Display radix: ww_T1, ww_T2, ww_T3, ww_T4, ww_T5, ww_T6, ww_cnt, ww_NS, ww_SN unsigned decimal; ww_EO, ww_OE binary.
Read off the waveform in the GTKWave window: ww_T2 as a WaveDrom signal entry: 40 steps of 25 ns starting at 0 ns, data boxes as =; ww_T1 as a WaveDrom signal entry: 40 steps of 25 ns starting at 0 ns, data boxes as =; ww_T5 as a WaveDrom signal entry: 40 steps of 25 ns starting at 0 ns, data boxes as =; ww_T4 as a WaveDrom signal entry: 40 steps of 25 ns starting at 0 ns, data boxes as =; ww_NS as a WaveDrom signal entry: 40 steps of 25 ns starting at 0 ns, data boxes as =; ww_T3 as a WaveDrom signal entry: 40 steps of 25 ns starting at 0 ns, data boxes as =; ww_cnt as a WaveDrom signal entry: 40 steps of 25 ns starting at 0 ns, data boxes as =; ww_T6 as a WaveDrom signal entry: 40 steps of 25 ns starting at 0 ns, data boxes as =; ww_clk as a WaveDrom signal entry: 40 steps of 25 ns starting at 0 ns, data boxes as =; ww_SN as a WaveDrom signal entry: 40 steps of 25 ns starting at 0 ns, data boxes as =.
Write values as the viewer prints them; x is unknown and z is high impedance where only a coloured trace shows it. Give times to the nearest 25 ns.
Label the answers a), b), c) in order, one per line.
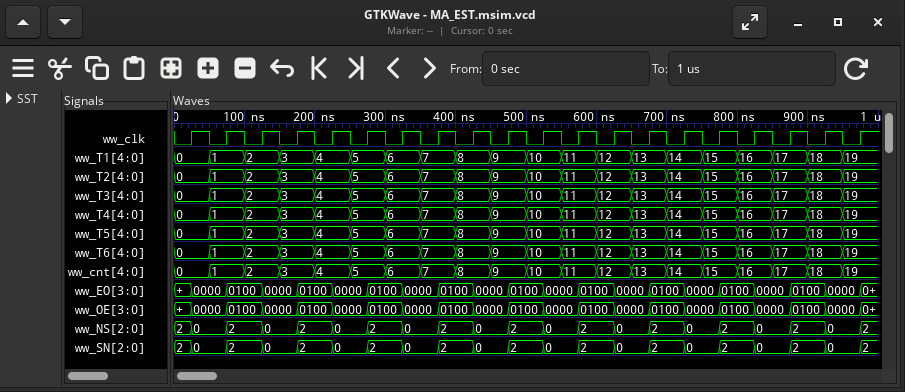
a) {name: 'ww_T2', wave: '=.=.=.=.=.=.=.=.=.=.=.=.=.=.=.=.=.=.=.=.', data: '0 1 2 3 4 5 6 7 8 9 10 11 12 13 14 15 16 17 18 19'}
b) {name: 'ww_T1', wave: '=.=.=.=.=.=.=.=.=.=.=.=.=.=.=.=.=.=.=.=.', data: '0 1 2 3 4 5 6 7 8 9 10 11 12 13 14 15 16 17 18 19'}
c) {name: 'ww_T5', wave: '=.=.=.=.=.=.=.=.=.=.=.=.=.=.=.=.=.=.=.=.', data: '0 1 2 3 4 5 6 7 8 9 10 11 12 13 14 15 16 17 18 19'}
d) {name: 'ww_T4', wave: '=.=.=.=.=.=.=.=.=.=.=.=.=.=.=.=.=.=.=.=.', data: '0 1 2 3 4 5 6 7 8 9 10 11 12 13 14 15 16 17 18 19'}
e) {name: 'ww_NS', wave: '==.=.=.=.=.=.=.=.=.=.=.=.=.=.=.=.=.=.=.=', data: '2 0 2 0 2 0 2 0 2 0 2 0 2 0 2 0 2 0 2 0 2'}
f) {name: 'ww_T3', wave: '=.=.=.=.=.=.=.=.=.=.=.=.=.=.=.=.=.=.=.=.', data: '0 1 2 3 4 5 6 7 8 9 10 11 12 13 14 15 16 17 18 19'}
g) {name: 'ww_cnt', wave: '=.=.=.=.=.=.=.=.=.=.=.=.=.=.=.=.=.=.=.=.', data: '0 1 2 3 4 5 6 7 8 9 10 11 12 13 14 15 16 17 18 19'}
h) {name: 'ww_T6', wave: '=.=.=.=.=.=.=.=.=.=.=.=.=.=.=.=.=.=.=.=.', data: '0 1 2 3 4 5 6 7 8 9 10 11 12 13 14 15 16 17 18 19'}
i) {name: 'ww_clk', wave: '0101010101010101010101010101010101010101'}
j) {name: 'ww_SN', wave: '==.=.=.=.=.=.=.=.=.=.=.=.=.=.=.=.=.=.=.=', data: '2 0 2 0 2 0 2 0 2 0 2 0 2 0 2 0 2 0 2 0 2'}
